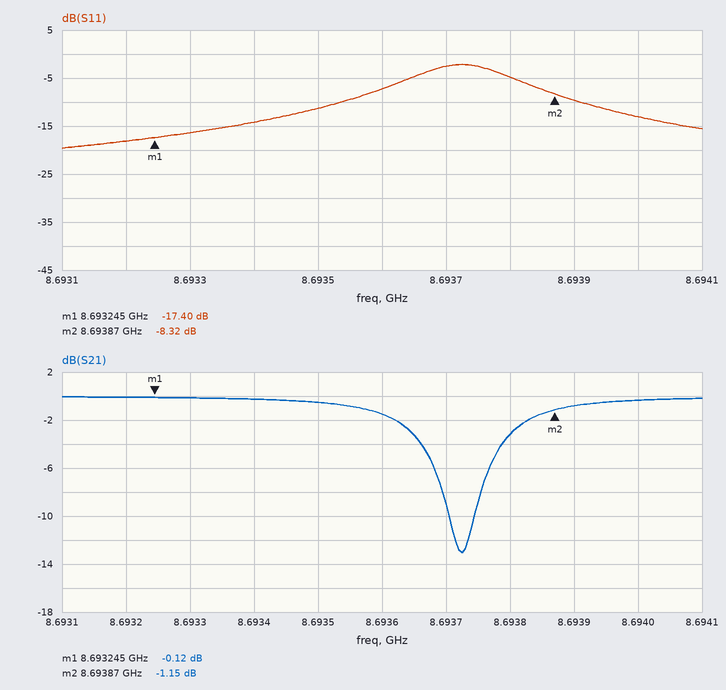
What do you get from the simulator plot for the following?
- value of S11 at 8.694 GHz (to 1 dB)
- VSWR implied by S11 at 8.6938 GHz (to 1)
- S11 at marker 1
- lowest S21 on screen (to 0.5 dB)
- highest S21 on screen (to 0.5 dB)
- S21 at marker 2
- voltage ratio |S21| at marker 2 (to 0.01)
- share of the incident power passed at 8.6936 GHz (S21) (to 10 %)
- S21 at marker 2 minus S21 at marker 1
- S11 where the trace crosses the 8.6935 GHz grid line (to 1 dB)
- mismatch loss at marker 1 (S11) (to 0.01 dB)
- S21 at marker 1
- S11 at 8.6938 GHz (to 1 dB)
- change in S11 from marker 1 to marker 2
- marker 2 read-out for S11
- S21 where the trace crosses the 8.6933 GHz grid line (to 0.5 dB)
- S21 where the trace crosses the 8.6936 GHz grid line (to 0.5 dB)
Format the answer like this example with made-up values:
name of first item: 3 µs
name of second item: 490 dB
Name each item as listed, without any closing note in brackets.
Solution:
value of S11 at 8.694 GHz: -13 dB
VSWR implied by S11 at 8.6938 GHz: 4
S11 at marker 1: -17.40 dB
lowest S21 on screen: -13.0 dB
highest S21 on screen: 0.0 dB
S21 at marker 2: -1.15 dB
voltage ratio |S21| at marker 2: 0.88
share of the incident power passed at 8.6936 GHz (S21): 70 %
S21 at marker 2 minus S21 at marker 1: -1.03 dB
S11 where the trace crosses the 8.6935 GHz grid line: -11 dB
mismatch loss at marker 1 (S11): 0.08 dB
S21 at marker 1: -0.12 dB
S11 at 8.6938 GHz: -5 dB
change in S11 from marker 1 to marker 2: 9.08 dB
marker 2 read-out for S11: -8.32 dB
S21 where the trace crosses the 8.6933 GHz grid line: 0.0 dB
S21 where the trace crosses the 8.6936 GHz grid line: -1.5 dB
